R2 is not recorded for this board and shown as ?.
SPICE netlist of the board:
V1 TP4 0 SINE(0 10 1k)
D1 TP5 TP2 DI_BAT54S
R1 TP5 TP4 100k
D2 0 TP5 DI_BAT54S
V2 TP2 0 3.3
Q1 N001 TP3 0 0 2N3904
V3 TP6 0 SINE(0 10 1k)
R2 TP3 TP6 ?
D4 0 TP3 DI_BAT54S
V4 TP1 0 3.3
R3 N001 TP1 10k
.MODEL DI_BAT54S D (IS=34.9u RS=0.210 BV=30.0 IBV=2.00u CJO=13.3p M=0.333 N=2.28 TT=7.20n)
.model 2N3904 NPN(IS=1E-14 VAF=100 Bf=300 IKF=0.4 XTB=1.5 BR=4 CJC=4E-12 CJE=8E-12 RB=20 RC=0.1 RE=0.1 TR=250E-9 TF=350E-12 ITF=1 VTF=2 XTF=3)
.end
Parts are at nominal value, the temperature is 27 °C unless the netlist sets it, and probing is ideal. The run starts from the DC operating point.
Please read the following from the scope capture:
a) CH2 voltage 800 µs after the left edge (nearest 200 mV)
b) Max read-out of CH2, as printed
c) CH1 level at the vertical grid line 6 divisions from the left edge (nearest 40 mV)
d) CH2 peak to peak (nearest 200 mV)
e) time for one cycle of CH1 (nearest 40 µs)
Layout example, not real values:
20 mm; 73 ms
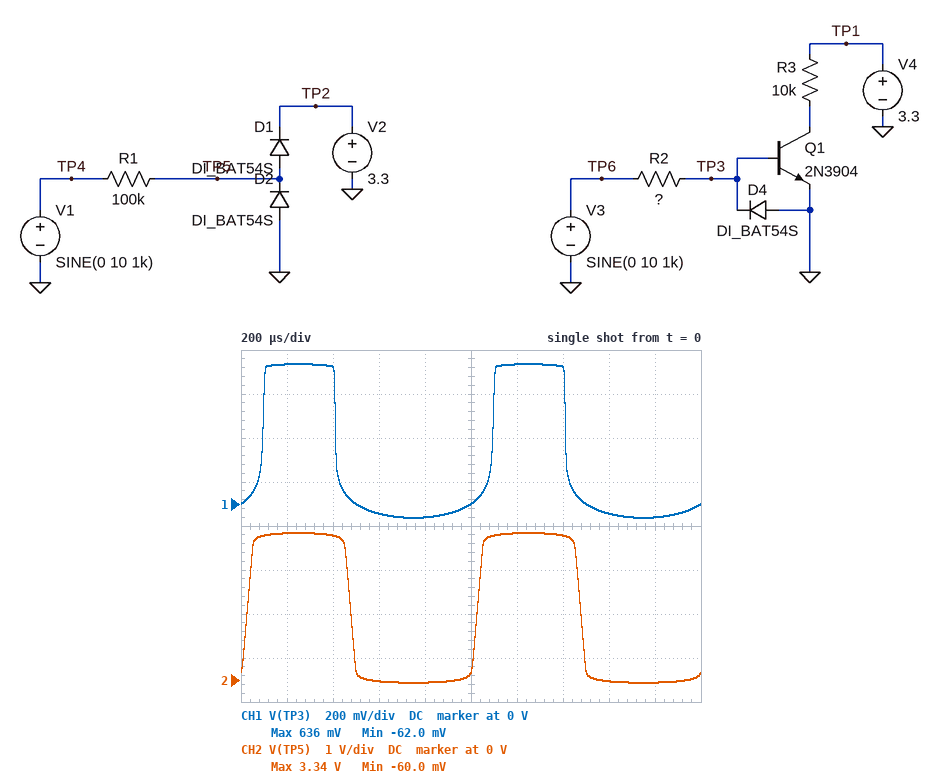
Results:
0 V; 3.34 V; 640 mV; 3.4 V; 1.00 ms
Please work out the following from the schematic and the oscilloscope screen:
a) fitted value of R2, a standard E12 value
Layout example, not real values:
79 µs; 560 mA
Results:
150 kΩ
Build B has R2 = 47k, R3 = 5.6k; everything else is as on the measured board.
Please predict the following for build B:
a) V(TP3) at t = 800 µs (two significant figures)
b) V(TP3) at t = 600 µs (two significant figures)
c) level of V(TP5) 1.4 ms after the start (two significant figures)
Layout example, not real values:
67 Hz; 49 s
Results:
-110 mV; -89 mV; 3.3 V
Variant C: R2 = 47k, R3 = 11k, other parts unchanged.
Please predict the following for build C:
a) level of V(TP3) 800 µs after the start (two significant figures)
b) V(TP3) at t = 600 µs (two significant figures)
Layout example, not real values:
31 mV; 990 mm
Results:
-110 mV; -89 mV
